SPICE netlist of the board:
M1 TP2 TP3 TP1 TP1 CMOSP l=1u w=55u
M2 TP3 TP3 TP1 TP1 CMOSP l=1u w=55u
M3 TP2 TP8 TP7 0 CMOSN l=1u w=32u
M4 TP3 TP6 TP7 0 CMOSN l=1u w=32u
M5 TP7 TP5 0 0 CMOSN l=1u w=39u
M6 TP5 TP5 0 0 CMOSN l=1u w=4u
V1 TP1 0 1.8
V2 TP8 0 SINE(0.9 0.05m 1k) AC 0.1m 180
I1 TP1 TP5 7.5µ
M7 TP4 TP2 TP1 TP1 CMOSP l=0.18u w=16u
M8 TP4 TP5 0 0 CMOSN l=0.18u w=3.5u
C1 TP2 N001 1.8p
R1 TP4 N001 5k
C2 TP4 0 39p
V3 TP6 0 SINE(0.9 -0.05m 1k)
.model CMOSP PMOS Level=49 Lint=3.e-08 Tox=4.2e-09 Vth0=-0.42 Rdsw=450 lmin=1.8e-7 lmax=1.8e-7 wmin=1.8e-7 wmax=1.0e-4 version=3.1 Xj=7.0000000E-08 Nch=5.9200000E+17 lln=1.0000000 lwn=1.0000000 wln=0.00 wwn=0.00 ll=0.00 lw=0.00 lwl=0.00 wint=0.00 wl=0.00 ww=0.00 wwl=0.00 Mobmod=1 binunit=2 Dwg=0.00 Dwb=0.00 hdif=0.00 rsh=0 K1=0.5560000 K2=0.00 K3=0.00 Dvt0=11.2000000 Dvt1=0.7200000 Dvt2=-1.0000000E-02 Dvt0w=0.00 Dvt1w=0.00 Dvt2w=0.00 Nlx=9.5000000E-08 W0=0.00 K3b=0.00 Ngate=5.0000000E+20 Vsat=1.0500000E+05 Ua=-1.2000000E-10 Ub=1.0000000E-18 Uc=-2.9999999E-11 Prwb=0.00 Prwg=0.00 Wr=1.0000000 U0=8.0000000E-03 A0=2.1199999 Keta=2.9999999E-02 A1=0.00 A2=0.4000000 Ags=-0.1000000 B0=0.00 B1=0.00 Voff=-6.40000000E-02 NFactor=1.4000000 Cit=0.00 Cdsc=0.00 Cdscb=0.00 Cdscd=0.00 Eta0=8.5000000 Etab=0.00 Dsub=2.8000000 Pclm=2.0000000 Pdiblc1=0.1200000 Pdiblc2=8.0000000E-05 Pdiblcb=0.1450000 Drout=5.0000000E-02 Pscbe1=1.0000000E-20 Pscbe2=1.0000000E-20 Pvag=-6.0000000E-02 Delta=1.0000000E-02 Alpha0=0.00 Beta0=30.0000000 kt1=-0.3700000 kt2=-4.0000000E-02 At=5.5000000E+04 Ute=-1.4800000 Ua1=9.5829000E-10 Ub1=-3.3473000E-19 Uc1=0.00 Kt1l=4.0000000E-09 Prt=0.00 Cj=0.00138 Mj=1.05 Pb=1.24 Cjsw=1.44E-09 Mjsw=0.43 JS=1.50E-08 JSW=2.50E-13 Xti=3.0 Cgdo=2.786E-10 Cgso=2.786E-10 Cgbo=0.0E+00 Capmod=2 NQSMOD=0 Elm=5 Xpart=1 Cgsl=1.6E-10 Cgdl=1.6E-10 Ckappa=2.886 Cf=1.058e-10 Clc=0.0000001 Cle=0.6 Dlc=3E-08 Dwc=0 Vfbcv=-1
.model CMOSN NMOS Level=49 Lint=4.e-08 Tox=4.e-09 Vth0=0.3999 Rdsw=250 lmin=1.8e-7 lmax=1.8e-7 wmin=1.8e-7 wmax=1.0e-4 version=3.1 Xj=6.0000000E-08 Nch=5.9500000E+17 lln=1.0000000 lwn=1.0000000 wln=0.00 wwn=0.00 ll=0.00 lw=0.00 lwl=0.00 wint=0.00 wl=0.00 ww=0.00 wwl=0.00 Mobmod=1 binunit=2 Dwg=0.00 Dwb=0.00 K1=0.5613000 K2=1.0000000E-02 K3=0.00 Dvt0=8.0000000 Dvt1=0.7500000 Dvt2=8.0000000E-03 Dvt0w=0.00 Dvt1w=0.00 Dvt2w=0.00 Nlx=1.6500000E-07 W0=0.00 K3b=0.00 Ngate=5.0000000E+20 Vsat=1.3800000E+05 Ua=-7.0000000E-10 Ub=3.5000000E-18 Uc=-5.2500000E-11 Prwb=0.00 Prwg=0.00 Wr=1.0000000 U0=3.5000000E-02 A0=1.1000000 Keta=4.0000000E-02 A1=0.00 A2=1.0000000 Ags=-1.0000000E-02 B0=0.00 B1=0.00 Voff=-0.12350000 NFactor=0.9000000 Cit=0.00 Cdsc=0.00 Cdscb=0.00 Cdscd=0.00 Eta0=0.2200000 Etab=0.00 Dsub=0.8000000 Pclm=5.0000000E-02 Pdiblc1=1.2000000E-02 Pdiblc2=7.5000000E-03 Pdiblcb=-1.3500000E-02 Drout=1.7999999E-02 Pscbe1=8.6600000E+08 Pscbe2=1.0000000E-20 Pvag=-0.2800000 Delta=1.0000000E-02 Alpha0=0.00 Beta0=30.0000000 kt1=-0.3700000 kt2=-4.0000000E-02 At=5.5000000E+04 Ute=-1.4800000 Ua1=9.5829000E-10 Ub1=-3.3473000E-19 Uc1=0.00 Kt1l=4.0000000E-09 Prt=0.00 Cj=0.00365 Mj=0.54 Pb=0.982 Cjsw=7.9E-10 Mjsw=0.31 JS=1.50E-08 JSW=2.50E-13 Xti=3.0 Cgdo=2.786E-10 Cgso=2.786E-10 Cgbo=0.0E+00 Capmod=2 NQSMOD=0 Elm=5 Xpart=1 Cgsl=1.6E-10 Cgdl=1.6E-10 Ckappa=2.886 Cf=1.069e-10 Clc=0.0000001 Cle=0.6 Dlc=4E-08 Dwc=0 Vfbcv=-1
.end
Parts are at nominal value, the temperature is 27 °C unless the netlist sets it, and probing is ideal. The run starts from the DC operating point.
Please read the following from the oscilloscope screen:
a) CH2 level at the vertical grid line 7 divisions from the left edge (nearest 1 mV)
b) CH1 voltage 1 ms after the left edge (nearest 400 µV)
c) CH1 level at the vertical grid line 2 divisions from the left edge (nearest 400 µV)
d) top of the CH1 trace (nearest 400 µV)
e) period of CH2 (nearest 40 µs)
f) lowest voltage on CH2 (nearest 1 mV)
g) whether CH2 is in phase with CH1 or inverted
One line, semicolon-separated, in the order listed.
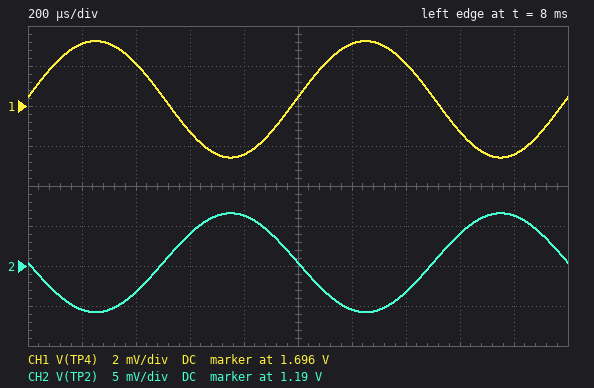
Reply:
1.187 V; 1.6964 V; 1.6980 V; 1.6992 V; 1.00 ms; 1.184 V; inverted
